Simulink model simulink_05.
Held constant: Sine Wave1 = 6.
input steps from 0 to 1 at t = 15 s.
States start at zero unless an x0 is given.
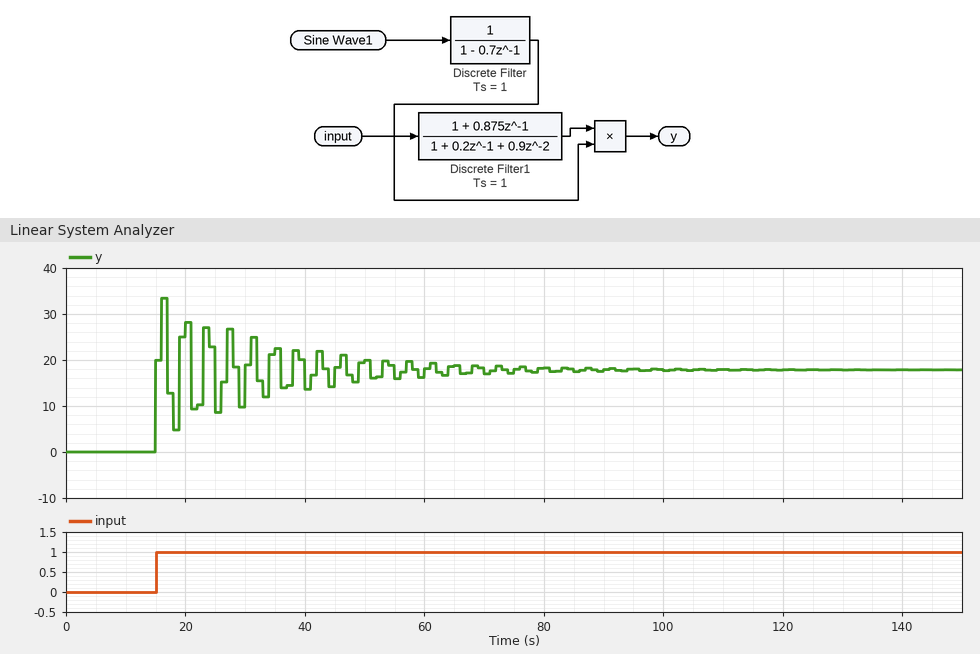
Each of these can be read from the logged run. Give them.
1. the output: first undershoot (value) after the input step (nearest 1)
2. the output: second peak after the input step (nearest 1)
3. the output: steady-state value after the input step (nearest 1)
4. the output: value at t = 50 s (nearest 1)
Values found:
5
28
18
20
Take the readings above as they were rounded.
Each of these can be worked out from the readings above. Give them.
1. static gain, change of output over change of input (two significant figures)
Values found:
18
